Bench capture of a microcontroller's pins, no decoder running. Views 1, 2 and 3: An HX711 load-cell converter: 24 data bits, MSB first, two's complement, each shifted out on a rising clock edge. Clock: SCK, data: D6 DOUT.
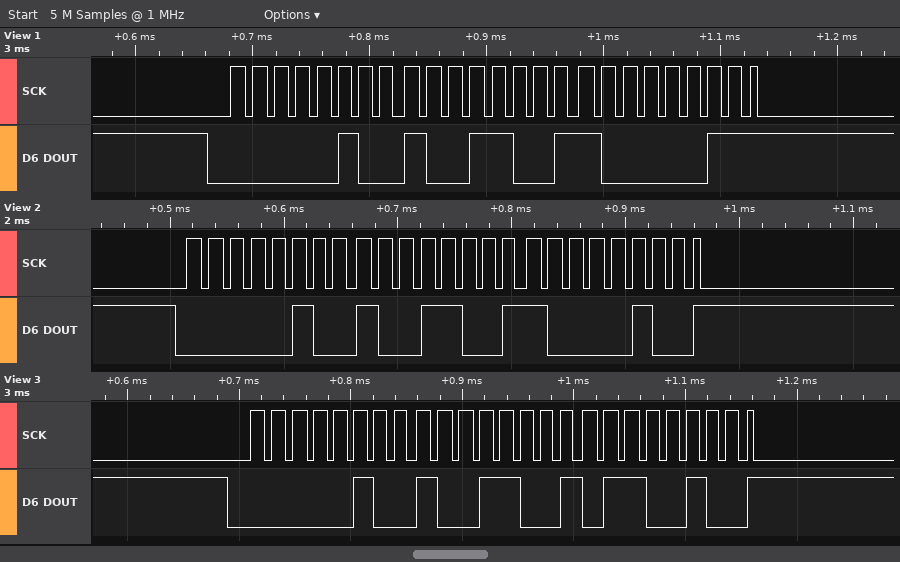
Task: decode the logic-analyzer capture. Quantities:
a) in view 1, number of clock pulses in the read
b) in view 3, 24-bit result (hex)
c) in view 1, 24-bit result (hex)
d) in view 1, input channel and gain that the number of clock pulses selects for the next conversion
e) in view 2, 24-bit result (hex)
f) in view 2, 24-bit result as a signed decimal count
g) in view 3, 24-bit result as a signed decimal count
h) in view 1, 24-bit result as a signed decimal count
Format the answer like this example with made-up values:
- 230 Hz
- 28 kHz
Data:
- 25
- 0x049964
- 0x049983
- channel A, gain 128
- 0x049984
- 301444
- 301412
- 301443
